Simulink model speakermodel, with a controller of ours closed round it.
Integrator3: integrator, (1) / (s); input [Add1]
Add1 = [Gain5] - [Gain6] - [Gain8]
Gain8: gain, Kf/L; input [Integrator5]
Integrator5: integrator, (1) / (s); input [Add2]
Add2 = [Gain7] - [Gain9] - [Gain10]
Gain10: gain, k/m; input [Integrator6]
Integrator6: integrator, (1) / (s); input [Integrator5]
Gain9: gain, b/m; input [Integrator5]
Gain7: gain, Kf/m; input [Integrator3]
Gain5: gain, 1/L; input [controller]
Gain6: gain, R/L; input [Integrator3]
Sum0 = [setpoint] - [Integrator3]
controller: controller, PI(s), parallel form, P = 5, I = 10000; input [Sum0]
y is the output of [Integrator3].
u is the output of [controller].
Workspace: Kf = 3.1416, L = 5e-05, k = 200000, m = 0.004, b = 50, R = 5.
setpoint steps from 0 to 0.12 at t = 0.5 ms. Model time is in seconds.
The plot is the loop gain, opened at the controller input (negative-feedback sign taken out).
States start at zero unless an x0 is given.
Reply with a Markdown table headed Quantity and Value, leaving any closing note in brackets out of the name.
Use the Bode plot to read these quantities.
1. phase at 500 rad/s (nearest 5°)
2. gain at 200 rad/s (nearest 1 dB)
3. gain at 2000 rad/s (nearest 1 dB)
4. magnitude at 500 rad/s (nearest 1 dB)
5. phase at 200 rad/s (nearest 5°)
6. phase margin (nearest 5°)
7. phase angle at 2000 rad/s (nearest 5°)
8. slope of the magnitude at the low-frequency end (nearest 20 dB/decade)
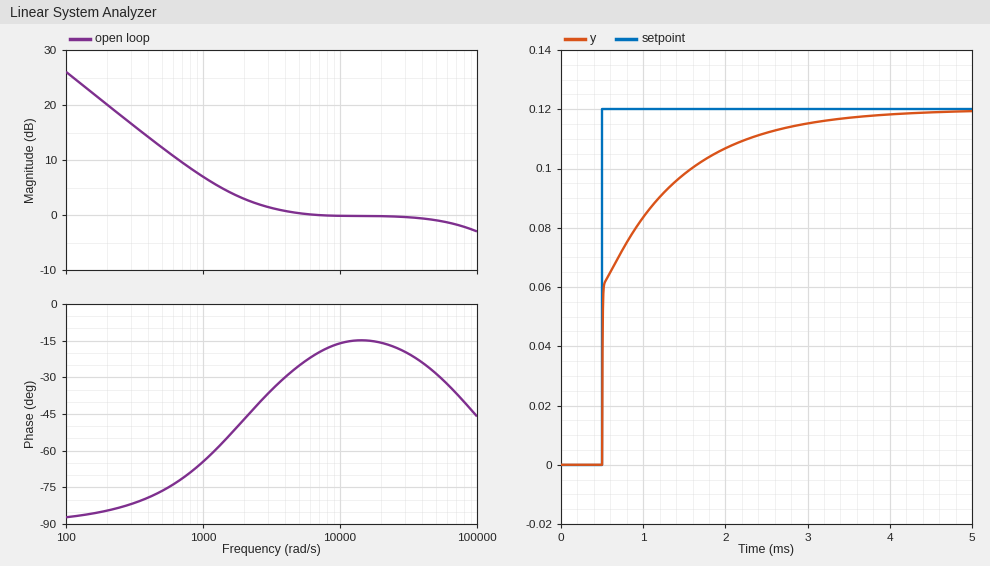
| Quantity | Value |
|---|---|
| phase at 500 rad/s | -75° |
| gain at 200 rad/s | 20 dB |
| gain at 2000 rad/s | 3 dB |
| magnitude at 500 rad/s | 12 dB |
| phase at 200 rad/s | -85° |
| phase margin | 160° |
| phase angle at 2000 rad/s | -45° |
| slope of the magnitude at the low-frequency end | -20 dB/decade |
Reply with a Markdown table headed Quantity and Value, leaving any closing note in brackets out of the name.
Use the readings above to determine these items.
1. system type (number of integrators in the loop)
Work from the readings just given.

| Quantity | Value |
|---|---|
| system type | 1 |
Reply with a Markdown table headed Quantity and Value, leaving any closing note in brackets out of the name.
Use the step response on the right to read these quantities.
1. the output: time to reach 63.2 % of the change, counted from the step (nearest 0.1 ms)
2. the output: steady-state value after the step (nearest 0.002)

| Quantity | Value |
|---|---|
| the output: time to reach 63.2 % of the change, counted from the step | 0.3 ms |
| the output: steady-state value after the step | 0.120 |
